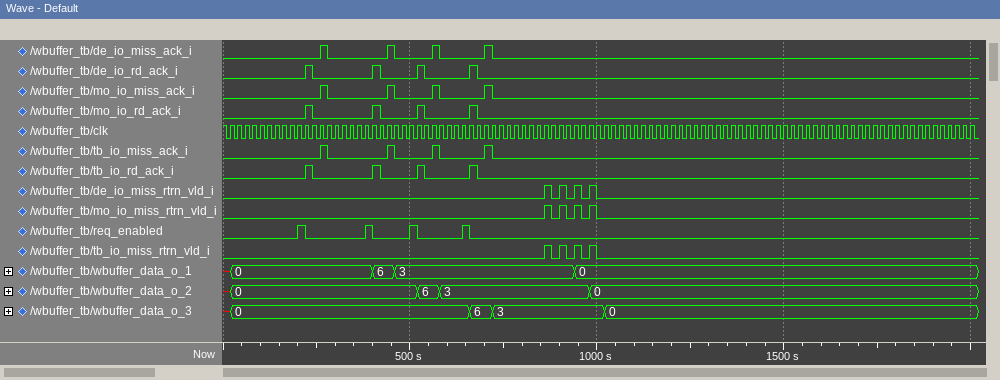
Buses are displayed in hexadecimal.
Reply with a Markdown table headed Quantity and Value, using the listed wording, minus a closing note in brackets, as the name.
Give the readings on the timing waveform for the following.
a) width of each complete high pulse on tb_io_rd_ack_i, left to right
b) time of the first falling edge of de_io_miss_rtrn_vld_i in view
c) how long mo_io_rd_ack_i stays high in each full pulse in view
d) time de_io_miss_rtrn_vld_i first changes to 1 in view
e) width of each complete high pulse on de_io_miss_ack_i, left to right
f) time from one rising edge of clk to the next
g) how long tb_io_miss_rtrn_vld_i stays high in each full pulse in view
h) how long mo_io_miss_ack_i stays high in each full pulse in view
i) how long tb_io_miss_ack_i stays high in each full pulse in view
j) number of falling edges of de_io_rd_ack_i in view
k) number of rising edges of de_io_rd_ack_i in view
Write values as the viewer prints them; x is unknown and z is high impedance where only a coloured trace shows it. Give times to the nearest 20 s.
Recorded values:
| Quantity | Value |
|---|---|
| width of each complete high pulse on tb_io_rd_ack_i, left to right | 20 s, 20 s, 20 s, 20 s |
| time of the first falling edge of de_io_miss_rtrn_vld_i in view | 880 s |
| how long mo_io_rd_ack_i stays high in each full pulse in view | 20 s, 20 s, 20 s, 20 s |
| time de_io_miss_rtrn_vld_i first changes to 1 in view | 860 s |
| width of each complete high pulse on de_io_miss_ack_i, left to right | 20 s, 20 s, 20 s, 20 s |
| time from one rising edge of clk to the next | 20 s |
| how long tb_io_miss_rtrn_vld_i stays high in each full pulse in view | 20 s, 20 s, 20 s, 20 s |
| how long mo_io_miss_ack_i stays high in each full pulse in view | 20 s, 20 s, 20 s, 20 s |
| how long tb_io_miss_ack_i stays high in each full pulse in view | 20 s, 20 s, 20 s, 20 s |
| number of falling edges of de_io_rd_ack_i in view | 4 |
| number of rising edges of de_io_rd_ack_i in view | 4 |
